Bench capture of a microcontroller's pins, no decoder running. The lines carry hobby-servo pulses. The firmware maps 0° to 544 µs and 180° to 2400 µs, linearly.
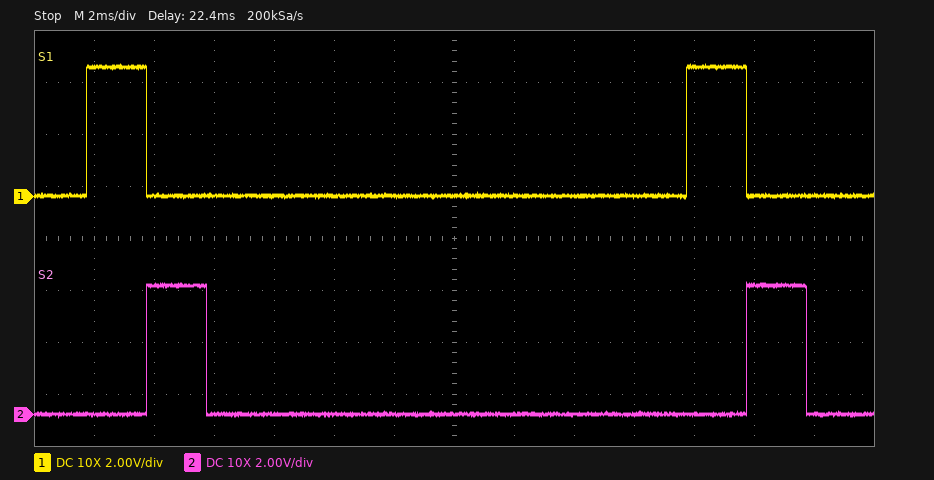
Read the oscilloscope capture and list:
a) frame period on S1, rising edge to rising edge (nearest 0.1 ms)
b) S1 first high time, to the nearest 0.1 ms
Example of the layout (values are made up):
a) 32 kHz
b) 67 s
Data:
a) 20.0 ms
b) 2.0 ms
